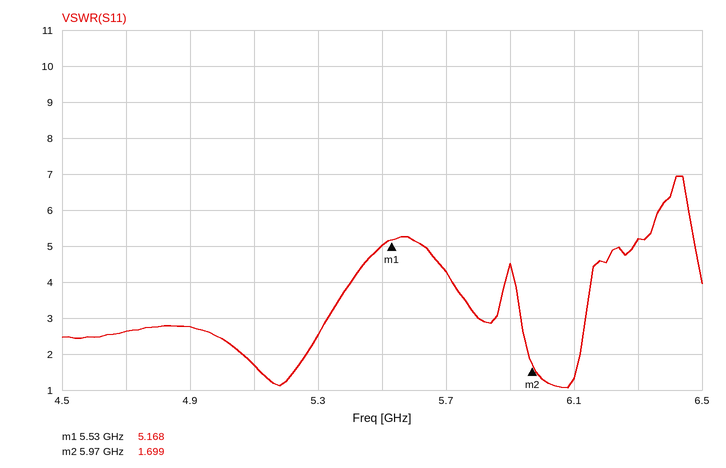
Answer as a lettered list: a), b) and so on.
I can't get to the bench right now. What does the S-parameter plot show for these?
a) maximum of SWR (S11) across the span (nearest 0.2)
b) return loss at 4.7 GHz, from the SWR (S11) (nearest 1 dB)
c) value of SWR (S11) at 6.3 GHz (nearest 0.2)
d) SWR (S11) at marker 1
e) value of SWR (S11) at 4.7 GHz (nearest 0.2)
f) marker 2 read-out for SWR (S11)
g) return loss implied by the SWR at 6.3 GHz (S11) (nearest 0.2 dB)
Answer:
a) 7.0
b) 7 dB
c) 5.2
d) 5.168
e) 2.6
f) 1.699
g) 3.4 dB
